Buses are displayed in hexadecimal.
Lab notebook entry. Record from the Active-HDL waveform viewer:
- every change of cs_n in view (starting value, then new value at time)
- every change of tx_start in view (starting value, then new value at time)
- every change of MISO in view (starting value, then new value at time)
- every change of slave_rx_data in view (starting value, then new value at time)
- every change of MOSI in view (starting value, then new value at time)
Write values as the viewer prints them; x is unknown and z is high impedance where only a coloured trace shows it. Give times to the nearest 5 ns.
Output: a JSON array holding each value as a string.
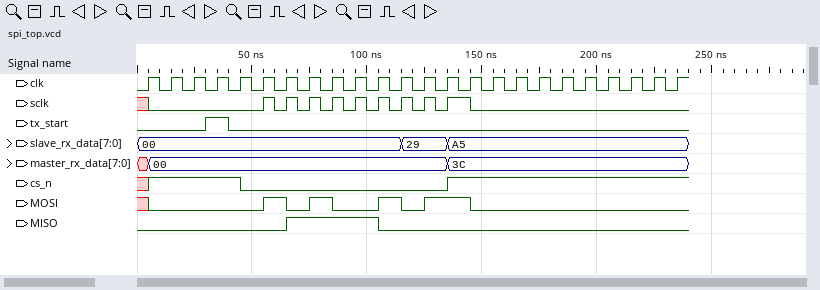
["x, 1 at 5 ns, 0 at 45 ns, 1 at 135 ns", "0, 1 at 30 ns, 0 at 40 ns", "0, 1 at 65 ns, 0 at 105 ns", "00, 29 at 115 ns, A5 at 135 ns", "x, 0 at 5 ns, 1 at 55 ns, 0 at 65 ns, 1 at 75 ns, 0 at 85 ns, 1 at 105 ns, 0 at 115 ns, 1 at 125 ns, 0 at 145 ns"]
